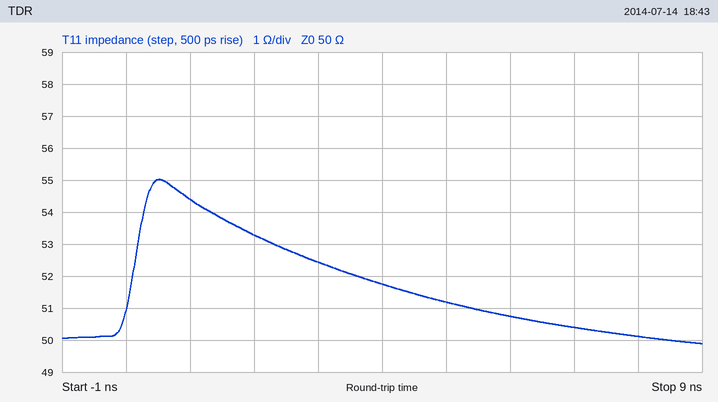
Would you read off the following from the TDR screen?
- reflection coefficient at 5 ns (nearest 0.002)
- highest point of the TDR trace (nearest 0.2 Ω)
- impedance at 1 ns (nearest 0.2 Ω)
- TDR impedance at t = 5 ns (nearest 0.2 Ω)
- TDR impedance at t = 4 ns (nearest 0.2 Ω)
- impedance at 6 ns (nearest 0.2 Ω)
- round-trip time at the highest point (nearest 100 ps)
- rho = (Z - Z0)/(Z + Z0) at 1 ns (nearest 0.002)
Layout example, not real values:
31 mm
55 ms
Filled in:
+0.012
55.0 Ω
54.4 Ω
51.2 Ω
51.8 Ω
50.8 Ω
500 ps
+0.042
